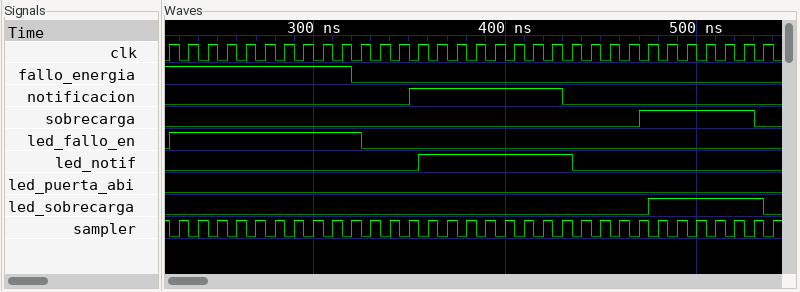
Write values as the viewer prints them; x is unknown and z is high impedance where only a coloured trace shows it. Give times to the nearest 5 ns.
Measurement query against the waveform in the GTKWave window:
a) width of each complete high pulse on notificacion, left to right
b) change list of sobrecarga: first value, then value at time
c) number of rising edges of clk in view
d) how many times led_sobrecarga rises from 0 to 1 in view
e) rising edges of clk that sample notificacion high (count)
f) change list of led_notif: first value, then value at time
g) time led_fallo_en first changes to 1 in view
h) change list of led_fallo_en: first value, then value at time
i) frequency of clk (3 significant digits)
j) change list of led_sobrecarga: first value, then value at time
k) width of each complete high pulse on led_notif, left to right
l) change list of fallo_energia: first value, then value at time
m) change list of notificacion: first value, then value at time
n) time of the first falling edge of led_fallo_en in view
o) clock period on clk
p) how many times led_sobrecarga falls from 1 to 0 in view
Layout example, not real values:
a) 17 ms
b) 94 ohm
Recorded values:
a) 80 ns
b) 0, 1 at 470 ns, 0 at 530 ns
c) 32
d) 1
e) 8
f) 0, 1 at 355 ns, 0 at 435 ns
g) 225 ns
h) 0, 1 at 225 ns, 0 at 325 ns
i) 100 MHz
j) 0, 1 at 475 ns, 0 at 535 ns
k) 80 ns
l) 1, 0 at 320 ns
m) 0, 1 at 350 ns, 0 at 430 ns
n) 325 ns
o) 10 ns
p) 1
